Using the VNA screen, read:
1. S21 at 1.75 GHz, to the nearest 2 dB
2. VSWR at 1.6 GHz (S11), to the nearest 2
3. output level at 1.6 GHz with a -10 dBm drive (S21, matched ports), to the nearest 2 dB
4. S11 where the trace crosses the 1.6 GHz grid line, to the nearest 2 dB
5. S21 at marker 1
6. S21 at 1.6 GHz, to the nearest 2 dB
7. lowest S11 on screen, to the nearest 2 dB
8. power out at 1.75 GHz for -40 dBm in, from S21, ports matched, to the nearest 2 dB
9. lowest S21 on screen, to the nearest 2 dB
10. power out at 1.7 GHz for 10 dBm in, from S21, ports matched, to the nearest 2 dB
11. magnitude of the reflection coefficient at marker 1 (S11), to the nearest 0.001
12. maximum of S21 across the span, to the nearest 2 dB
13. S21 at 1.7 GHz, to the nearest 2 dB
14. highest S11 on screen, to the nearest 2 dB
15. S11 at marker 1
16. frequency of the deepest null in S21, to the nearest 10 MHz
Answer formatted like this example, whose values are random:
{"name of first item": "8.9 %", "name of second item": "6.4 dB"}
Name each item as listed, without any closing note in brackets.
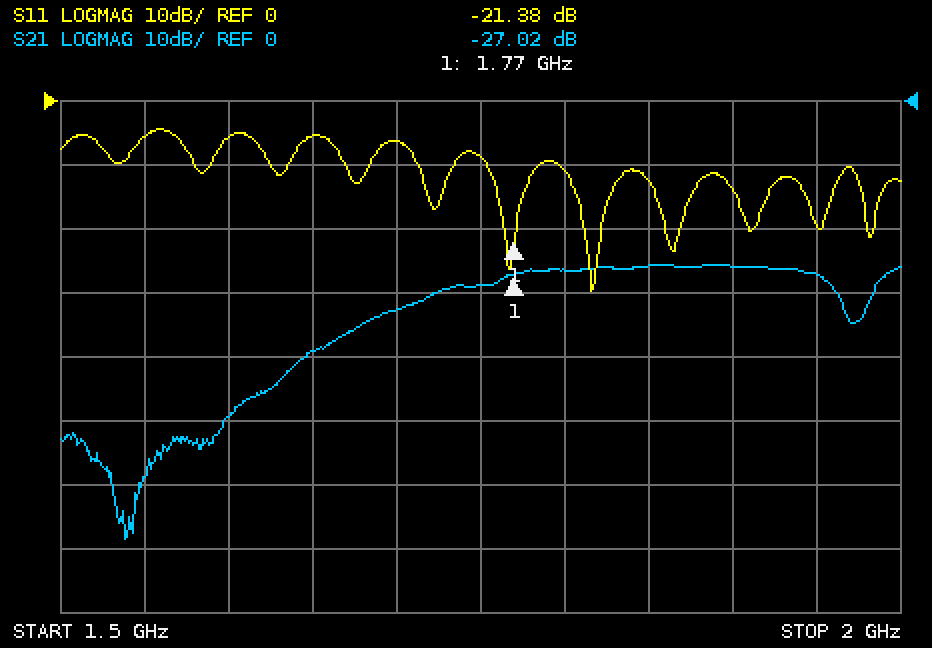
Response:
{"S21 at 1.75 GHz, to the nearest 2 dB": "-28 dB", "VSWR at 1.6 GHz (S11), to the nearest 2": "4", "output level at 1.6 GHz with a -10 dBm drive (S21, matched ports), to the nearest 2 dB": "-60 dBm", "S11 where the trace crosses the 1.6 GHz grid line, to the nearest 2 dB": "-6 dB", "S21 at marker 1": "-27.02 dB", "S21 at 1.6 GHz, to the nearest 2 dB": "-50 dB", "lowest S11 on screen, to the nearest 2 dB": "-30 dB", "power out at 1.75 GHz for -40 dBm in, from S21, ports matched, to the nearest 2 dB": "-68 dBm", "lowest S21 on screen, to the nearest 2 dB": "-68 dB", "power out at 1.7 GHz for 10 dBm in, from S21, ports matched, to the nearest 2 dB": "-22 dBm", "magnitude of the reflection coefficient at marker 1 (S11), to the nearest 0.001": "0.085", "maximum of S21 across the span, to the nearest 2 dB": "-26 dB", "S21 at 1.7 GHz, to the nearest 2 dB": "-32 dB", "highest S11 on screen, to the nearest 2 dB": "-4 dB", "S11 at marker 1": "-21.38 dB", "frequency of the deepest null in S21, to the nearest 10 MHz": "1.54 GHz"}
